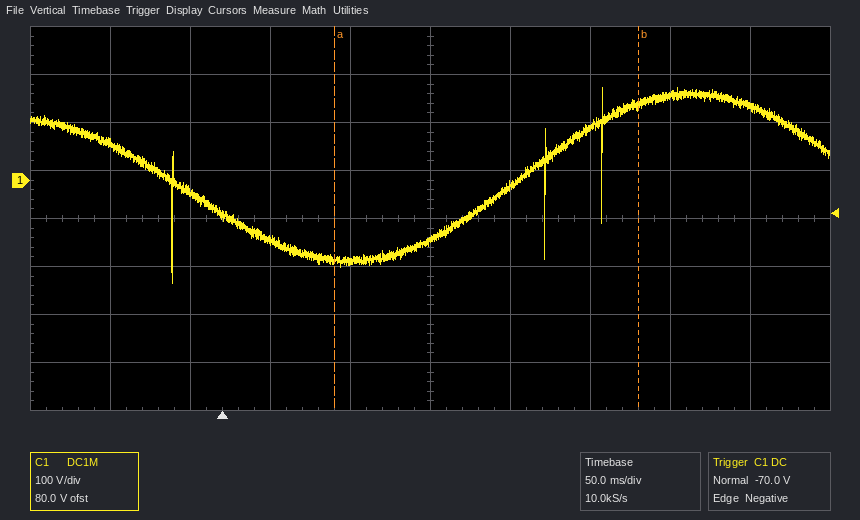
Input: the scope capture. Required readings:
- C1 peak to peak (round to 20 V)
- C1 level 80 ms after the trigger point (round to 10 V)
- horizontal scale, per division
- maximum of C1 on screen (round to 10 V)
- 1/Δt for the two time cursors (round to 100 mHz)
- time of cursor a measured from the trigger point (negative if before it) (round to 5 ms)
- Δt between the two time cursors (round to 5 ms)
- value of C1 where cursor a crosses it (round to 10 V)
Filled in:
400 V
-170 V
50 ms
190 V
5.3 Hz
+70 ms
190 ms
-170 V
